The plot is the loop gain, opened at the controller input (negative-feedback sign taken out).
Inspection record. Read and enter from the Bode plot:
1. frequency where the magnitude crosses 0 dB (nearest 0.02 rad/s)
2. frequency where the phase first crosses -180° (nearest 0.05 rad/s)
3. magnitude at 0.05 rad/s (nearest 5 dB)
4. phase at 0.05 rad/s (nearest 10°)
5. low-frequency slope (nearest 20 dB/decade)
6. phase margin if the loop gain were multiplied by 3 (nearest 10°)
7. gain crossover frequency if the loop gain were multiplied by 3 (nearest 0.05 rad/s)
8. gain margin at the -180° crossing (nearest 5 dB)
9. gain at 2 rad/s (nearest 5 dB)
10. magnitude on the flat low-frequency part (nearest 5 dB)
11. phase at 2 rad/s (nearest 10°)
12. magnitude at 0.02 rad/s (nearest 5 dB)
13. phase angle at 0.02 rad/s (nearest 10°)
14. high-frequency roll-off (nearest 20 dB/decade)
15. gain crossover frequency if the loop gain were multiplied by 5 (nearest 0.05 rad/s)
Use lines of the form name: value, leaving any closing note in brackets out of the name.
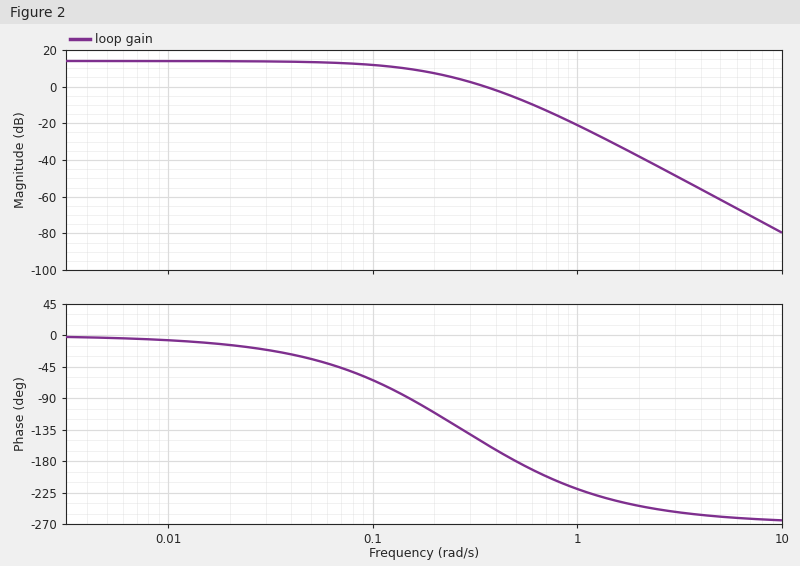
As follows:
frequency where the magnitude crosses 0 dB: 0.36 rad/s
frequency where the phase first crosses -180°: 0.50 rad/s
magnitude at 0.05 rad/s: 15 dB
phase at 0.05 rad/s: -30°
low-frequency slope: 0 dB/decade
phase margin if the loop gain were multiplied by 3: -10°
gain crossover frequency if the loop gain were multiplied by 3: 0.60 rad/s
gain margin at the -180° crossing: 5 dB
gain at 2 rad/s: -40 dB
magnitude on the flat low-frequency part: 15 dB
phase at 2 rad/s: -240°
magnitude at 0.02 rad/s: 15 dB
phase angle at 0.02 rad/s: -10°
high-frequency roll-off: -60 dB/decade
gain crossover frequency if the loop gain were multiplied by 5: 0.75 rad/s
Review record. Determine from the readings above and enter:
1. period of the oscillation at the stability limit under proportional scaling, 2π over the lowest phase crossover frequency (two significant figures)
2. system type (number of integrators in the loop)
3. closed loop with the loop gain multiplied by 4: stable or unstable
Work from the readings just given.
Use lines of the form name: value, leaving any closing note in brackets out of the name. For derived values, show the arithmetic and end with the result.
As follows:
period of the oscillation at the stability limit under proportional scaling, 2π over the lowest phase crossover frequency: 2π / 0.5 = 13 s
system type: 0
closed loop with the loop gain multiplied by 4: stable or unstable: unstable
